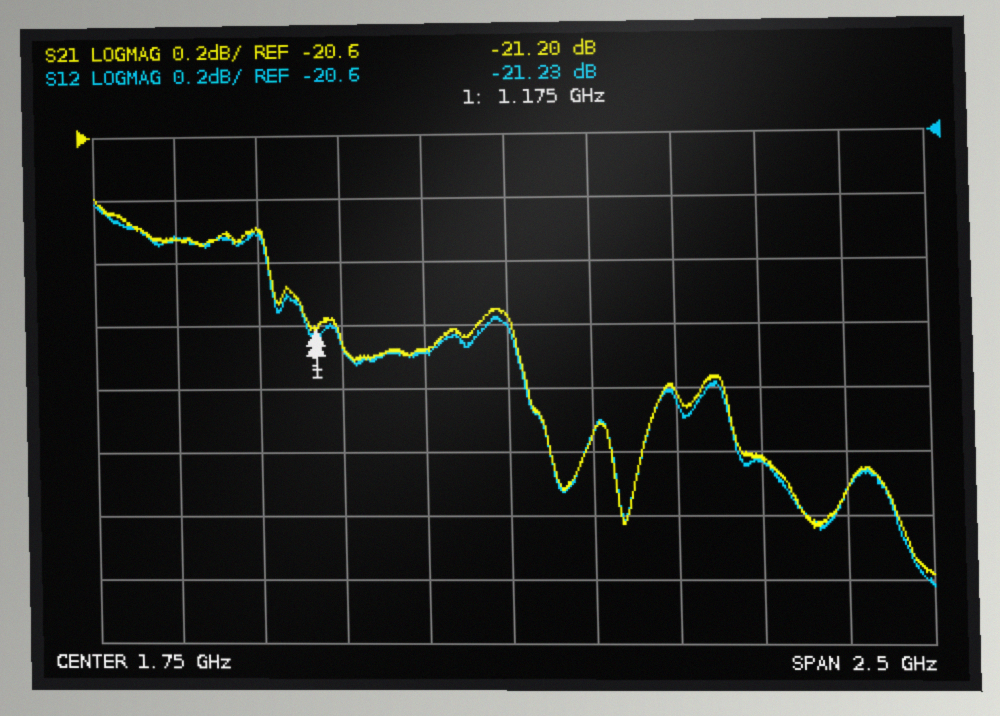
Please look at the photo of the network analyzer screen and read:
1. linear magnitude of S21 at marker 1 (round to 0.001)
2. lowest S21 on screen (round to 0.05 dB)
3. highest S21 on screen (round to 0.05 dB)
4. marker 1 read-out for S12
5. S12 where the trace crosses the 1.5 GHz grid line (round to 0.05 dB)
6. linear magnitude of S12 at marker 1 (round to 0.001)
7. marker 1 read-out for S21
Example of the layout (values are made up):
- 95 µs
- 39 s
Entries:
- 0.087
- -22.00 dB
- -20.80 dB
- -21.23 dB
- -21.30 dB
- 0.087
- -21.20 dB
